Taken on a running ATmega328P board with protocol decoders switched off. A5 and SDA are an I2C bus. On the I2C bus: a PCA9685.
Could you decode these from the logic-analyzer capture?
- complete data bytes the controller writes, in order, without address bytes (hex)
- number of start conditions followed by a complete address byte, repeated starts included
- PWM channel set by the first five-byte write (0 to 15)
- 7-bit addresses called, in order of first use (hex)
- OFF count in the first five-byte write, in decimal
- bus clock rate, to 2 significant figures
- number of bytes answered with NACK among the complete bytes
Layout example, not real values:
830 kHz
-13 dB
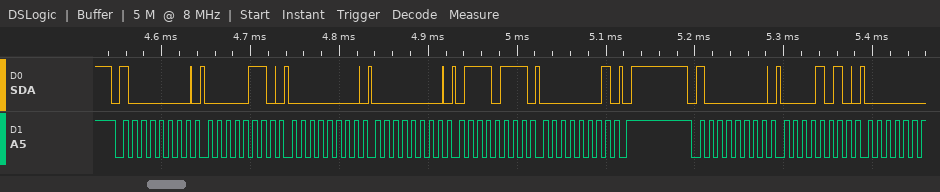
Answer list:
06 00 00 77 01 0A
2
0
0x40
375
100 kHz
0
